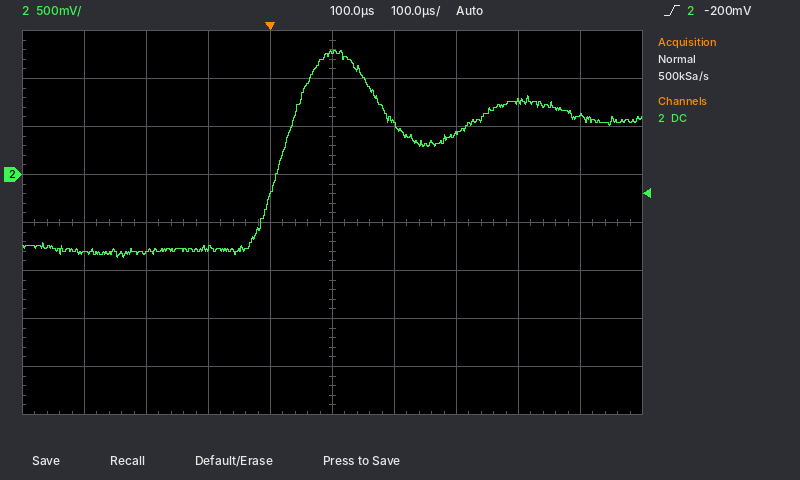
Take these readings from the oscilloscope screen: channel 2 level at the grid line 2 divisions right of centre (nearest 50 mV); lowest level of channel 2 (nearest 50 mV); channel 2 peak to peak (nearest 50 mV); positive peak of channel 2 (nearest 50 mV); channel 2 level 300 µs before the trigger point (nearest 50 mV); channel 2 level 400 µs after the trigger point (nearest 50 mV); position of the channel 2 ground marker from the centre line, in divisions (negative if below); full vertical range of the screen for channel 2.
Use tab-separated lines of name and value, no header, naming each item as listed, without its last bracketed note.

channel 2 level at the grid line 2 divisions right of centre	400 mV
lowest level of channel 2	-850 mV
channel 2 peak to peak	2.15 V
positive peak of channel 2	1.30 V
channel 2 level 300 µs before the trigger point	-800 mV
channel 2 level 400 µs after the trigger point	750 mV
position of the channel 2 ground marker from the centre line, in divisions	+1.0 div
full vertical range of the screen for channel 2	4 V
